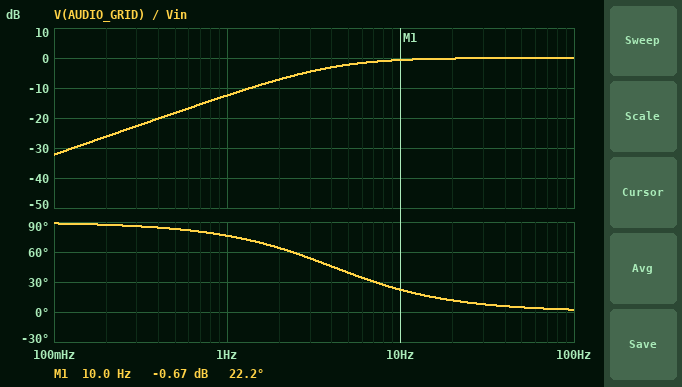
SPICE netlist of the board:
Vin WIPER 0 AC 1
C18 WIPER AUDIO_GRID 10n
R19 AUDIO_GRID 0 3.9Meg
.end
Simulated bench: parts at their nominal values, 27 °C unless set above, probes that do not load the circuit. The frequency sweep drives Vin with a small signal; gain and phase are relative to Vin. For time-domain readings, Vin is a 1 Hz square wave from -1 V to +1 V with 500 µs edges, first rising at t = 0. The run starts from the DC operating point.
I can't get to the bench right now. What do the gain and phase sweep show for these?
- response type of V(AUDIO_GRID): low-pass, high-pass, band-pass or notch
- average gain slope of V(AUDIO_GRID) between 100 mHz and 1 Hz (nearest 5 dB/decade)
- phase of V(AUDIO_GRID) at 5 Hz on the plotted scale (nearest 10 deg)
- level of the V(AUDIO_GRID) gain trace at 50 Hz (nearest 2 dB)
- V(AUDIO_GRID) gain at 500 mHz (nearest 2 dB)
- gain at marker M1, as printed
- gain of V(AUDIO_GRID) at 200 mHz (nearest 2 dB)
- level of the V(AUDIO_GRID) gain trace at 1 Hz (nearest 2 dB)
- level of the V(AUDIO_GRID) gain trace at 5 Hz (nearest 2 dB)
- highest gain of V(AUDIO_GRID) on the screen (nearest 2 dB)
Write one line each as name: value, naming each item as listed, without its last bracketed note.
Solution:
response type of V(AUDIO_GRID): low-pass, high-pass, band-pass or notch: high-pass
average gain slope of V(AUDIO_GRID) between 100 mHz and 1 Hz: 20 dB/decade
phase of V(AUDIO_GRID) at 5 Hz on the plotted scale: 40 deg
level of the V(AUDIO_GRID) gain trace at 50 Hz: 0 dB
V(AUDIO_GRID) gain at 500 mHz: -18 dB
gain at marker M1, as printed: -0.67 dB
gain of V(AUDIO_GRID) at 200 mHz: -26 dB
level of the V(AUDIO_GRID) gain trace at 1 Hz: -12 dB
level of the V(AUDIO_GRID) gain trace at 5 Hz: -2 dB
highest gain of V(AUDIO_GRID) on the screen: 0 dB
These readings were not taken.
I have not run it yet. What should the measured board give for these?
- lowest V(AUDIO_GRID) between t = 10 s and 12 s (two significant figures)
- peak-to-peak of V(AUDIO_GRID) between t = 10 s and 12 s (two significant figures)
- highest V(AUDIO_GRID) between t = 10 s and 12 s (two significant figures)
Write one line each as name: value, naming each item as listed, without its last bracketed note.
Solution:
lowest V(AUDIO_GRID) between t = 10 s and 12 s: -2.0 V
peak-to-peak of V(AUDIO_GRID) between t = 10 s and 12 s: 4.0 V
highest V(AUDIO_GRID) between t = 10 s and 12 s: 2.0 V
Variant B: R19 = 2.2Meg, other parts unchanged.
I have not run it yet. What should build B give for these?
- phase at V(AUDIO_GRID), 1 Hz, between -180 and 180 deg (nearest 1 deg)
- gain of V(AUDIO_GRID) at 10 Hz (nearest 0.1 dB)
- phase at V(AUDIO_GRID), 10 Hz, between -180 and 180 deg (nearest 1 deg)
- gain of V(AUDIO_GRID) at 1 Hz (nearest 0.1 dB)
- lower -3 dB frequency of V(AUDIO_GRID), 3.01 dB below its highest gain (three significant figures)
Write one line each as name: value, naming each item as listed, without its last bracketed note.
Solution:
phase at V(AUDIO_GRID), 1 Hz, between -180 and 180 deg: 82 deg
gain of V(AUDIO_GRID) at 10 Hz: -1.8 dB
phase at V(AUDIO_GRID), 10 Hz, between -180 and 180 deg: 36 deg
gain of V(AUDIO_GRID) at 1 Hz: -17.3 dB
lower -3 dB frequency of V(AUDIO_GRID), 3.01 dB below its highest gain: 7.23 Hz
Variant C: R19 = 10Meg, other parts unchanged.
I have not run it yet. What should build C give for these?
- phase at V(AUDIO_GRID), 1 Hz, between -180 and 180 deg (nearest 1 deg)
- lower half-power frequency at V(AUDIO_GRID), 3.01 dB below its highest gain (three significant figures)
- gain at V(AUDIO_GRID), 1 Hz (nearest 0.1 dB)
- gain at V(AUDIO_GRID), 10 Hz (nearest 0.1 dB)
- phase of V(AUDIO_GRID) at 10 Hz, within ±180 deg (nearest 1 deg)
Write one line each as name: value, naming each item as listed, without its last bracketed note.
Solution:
phase at V(AUDIO_GRID), 1 Hz, between -180 and 180 deg: 58 deg
lower half-power frequency at V(AUDIO_GRID), 3.01 dB below its highest gain: 1.59 Hz
gain at V(AUDIO_GRID), 1 Hz: -5.5 dB
gain at V(AUDIO_GRID), 10 Hz: -0.1 dB
phase of V(AUDIO_GRID) at 10 Hz, within ±180 deg: 9 deg
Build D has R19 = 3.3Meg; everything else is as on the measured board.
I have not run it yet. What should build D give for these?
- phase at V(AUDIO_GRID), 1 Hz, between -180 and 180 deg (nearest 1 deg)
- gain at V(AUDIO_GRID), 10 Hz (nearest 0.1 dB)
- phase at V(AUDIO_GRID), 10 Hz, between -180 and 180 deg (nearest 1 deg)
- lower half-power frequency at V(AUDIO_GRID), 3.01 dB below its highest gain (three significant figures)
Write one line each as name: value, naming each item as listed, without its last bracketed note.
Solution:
phase at V(AUDIO_GRID), 1 Hz, between -180 and 180 deg: 78 deg
gain at V(AUDIO_GRID), 10 Hz: -0.9 dB
phase at V(AUDIO_GRID), 10 Hz, between -180 and 180 deg: 26 deg
lower half-power frequency at V(AUDIO_GRID), 3.01 dB below its highest gain: 4.82 Hz
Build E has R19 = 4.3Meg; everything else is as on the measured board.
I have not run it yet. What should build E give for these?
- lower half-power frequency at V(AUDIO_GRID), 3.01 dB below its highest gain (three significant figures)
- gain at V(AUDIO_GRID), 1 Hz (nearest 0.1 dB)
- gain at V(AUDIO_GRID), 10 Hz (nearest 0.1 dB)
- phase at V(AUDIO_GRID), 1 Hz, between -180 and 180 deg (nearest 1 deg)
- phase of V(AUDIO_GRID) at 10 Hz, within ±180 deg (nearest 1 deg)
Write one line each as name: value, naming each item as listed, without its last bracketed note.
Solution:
lower half-power frequency at V(AUDIO_GRID), 3.01 dB below its highest gain: 3.70 Hz
gain at V(AUDIO_GRID), 1 Hz: -11.7 dB
gain at V(AUDIO_GRID), 10 Hz: -0.6 dB
phase at V(AUDIO_GRID), 1 Hz, between -180 and 180 deg: 75 deg
phase of V(AUDIO_GRID) at 10 Hz, within ±180 deg: 20 deg
